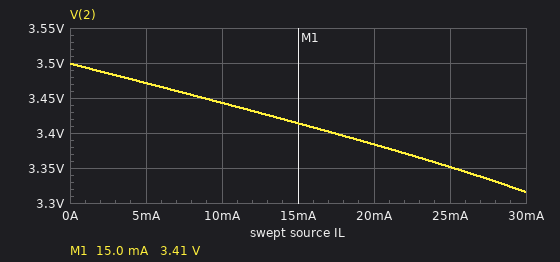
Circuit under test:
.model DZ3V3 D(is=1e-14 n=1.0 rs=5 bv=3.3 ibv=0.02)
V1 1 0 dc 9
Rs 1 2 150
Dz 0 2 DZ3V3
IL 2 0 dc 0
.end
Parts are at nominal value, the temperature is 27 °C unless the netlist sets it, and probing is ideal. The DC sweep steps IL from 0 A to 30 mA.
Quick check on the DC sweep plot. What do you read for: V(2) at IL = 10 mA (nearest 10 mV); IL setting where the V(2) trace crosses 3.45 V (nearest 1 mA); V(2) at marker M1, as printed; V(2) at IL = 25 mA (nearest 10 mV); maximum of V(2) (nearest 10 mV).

3.44 V
9 mA
3.41 V
3.35 V
3.50 V
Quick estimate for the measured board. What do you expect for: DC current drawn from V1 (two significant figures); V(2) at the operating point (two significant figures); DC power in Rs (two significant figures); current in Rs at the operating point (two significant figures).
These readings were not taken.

37 mA
3.5 V
200 mW
37 mA
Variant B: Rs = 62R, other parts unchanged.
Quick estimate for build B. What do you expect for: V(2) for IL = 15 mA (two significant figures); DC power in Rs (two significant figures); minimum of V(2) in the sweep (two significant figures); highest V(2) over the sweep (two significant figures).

3.7 V
440 mW
3.6 V
3.8 V
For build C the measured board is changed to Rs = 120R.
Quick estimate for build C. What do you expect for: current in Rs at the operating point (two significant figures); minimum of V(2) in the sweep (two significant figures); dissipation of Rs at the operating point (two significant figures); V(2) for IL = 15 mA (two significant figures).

45 mA
3.4 V
250 mW
3.5 V
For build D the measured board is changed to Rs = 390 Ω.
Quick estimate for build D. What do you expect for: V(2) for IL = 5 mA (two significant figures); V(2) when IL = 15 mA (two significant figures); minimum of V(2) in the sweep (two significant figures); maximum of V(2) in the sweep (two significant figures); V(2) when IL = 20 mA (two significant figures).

3.3 V
3.1 V
-720 mV
3.4 V
1.2 V
